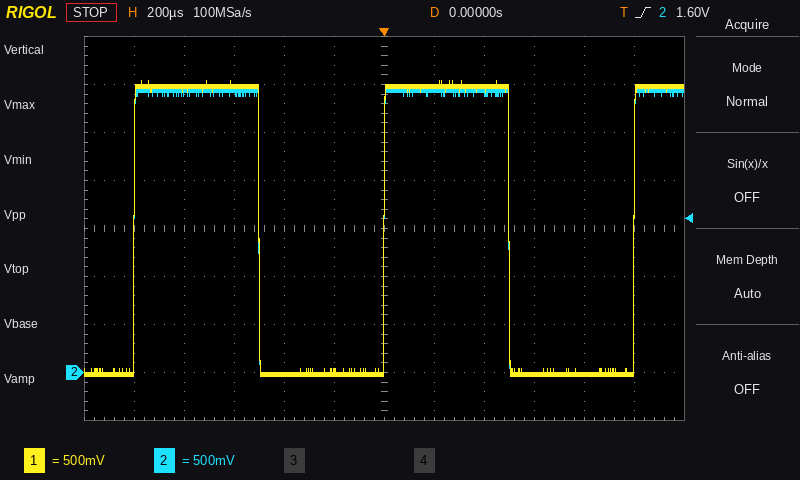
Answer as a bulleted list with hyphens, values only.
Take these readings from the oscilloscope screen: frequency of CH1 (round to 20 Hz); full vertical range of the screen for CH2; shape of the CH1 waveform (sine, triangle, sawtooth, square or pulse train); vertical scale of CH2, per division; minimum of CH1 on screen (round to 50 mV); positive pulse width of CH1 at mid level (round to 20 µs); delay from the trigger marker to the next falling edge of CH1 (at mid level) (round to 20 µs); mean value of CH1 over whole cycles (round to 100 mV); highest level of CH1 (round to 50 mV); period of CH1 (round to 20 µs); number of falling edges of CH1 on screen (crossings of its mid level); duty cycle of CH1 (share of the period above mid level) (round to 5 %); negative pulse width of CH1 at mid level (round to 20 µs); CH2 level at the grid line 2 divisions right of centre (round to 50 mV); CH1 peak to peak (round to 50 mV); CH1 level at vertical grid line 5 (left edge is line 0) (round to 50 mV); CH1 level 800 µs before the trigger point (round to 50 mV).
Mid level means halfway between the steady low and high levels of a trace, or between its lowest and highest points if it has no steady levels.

- 1.00 kHz
- 4 V
- square
- 500 mV
- -50 mV
- 500 µs
- 500 µs
- 1.5 V
- 3.05 V
- 1.00 ms
- 2
- 50 %
- 500 µs
- 2.90 V
- 3.10 V
- 0 mV
- 2.95 V
